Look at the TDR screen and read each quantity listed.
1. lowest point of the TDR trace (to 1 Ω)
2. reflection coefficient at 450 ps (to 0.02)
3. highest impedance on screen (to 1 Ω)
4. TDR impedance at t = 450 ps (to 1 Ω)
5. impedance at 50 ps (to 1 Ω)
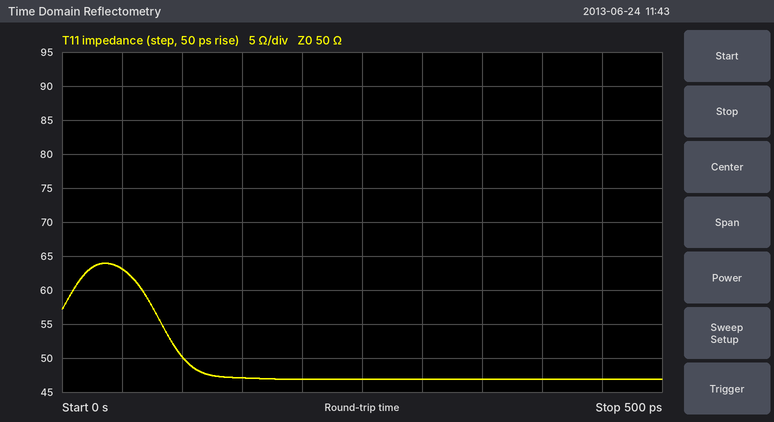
47 Ω
-0.04
64 Ω
47 Ω
63 Ω
